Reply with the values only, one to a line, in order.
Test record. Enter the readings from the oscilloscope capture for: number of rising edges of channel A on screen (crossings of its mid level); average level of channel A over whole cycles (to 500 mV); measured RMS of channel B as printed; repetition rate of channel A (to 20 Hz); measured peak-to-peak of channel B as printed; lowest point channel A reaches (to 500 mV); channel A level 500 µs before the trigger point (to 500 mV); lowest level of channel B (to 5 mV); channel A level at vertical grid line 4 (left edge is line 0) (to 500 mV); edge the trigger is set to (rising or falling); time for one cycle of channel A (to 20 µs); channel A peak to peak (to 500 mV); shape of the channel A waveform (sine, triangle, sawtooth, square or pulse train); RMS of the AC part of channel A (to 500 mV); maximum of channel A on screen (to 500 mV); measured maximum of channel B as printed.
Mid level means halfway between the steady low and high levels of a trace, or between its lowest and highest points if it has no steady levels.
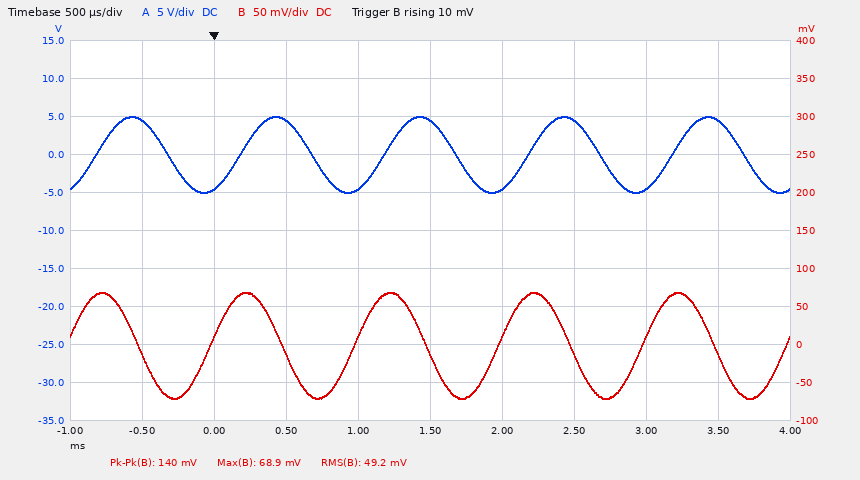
5
0.0 V
49.2 mV
1.00 kHz
140 mV
-5.0 V
4.5 V
-70 mV
-4.5 V
rising
1.00 ms
10.0 V
sine
3.5 V
5.0 V
68.9 mV
